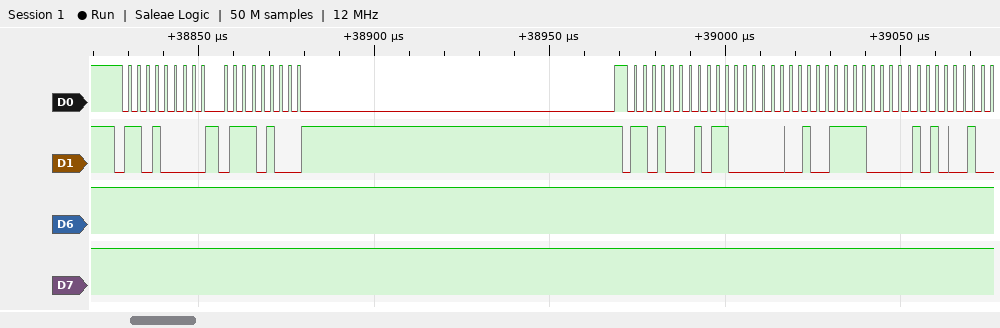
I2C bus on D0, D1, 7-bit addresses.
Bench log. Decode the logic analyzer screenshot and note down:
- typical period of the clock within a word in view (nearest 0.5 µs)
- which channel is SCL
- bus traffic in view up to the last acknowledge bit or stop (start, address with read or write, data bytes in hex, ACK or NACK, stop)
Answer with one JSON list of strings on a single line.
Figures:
["2.5 µs", "D0", "start, address 68 write ACK, 74 ACK, repeated start, address 68 read ACK, C0 ACK, 4F ACK, 0A ACK"]
